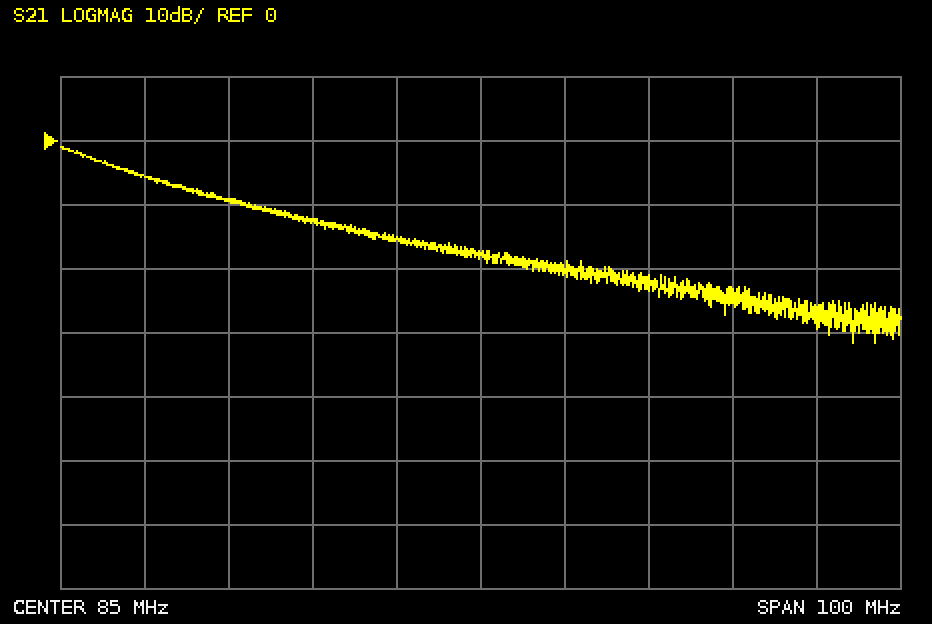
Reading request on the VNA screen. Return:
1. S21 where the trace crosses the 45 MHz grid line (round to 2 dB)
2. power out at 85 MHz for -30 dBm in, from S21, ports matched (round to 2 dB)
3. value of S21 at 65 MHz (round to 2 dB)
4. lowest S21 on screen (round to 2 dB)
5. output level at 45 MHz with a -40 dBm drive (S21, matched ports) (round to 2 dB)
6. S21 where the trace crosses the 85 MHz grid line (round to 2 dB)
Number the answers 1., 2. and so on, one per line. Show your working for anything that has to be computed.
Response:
1. -6 dB
2. -30 dBm + (-18 dB) = -48 dBm
3. -12 dB
4. -32 dB
5. -40 dBm + (-6 dB) = -46 dBm
6. -18 dB
